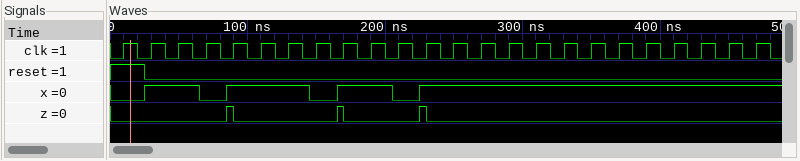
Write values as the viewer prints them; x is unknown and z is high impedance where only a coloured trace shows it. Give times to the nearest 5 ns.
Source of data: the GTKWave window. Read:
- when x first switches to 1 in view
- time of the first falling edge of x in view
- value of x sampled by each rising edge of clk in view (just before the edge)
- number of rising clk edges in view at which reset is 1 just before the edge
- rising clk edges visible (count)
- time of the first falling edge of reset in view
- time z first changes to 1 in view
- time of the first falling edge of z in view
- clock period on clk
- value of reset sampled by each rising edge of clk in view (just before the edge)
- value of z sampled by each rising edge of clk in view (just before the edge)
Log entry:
25 ns
65 ns
0 1 1 0 1 1 1 0 1 1 0 1 1 1 1 1 1 1 1 1 1 1 1 1
1
24
25 ns
85 ns
90 ns
20 ns
1 0 0 0 0 0 0 0 0 0 0 0 0 0 0 0 0 0 0 0 0 0 0 0
0 0 0 0 1 0 0 0 1 0 0 1 0 0 0 0 0 0 0 0 0 0 0 0
